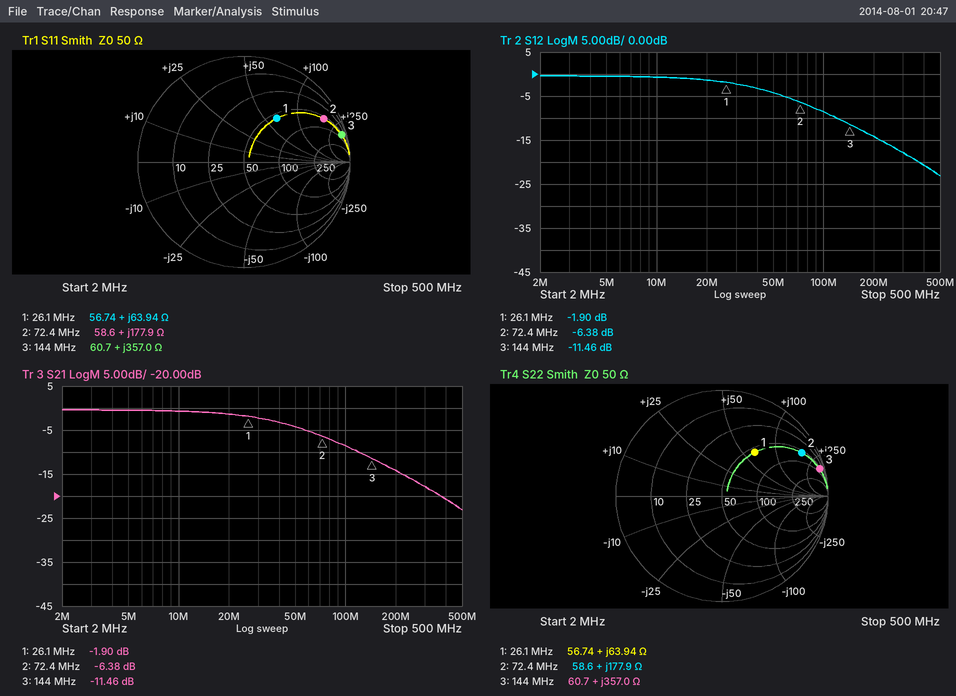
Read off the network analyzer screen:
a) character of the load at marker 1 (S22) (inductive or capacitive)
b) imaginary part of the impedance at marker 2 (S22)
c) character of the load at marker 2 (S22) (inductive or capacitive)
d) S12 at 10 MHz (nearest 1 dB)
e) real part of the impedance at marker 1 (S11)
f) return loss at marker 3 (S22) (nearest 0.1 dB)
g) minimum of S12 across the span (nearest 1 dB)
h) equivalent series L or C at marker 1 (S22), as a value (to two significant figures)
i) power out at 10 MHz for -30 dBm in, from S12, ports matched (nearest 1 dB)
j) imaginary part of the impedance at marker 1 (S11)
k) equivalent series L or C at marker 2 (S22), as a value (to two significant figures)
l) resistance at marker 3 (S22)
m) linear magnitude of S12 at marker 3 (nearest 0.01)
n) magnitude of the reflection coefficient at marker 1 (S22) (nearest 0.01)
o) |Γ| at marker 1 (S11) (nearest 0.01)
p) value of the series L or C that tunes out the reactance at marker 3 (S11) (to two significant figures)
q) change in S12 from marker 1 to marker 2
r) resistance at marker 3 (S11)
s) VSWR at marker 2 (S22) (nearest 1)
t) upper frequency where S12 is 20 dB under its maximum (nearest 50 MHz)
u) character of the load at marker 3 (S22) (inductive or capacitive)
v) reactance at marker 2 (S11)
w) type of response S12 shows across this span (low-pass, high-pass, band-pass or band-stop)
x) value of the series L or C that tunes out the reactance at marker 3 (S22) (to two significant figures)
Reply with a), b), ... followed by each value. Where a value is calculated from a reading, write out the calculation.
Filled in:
a) inductive
b) +177.9 Ω
c) inductive
d) -1 dB
e) 56.74 Ω
f) 0.4 dB
g) -23 dB
h) L = 63.94 Ω/(2π × 26.1 MHz) ≈ 390 nH
i) -30 dBm + (-1 dB) = -31 dBm
j) +63.94 Ω
k) L = 177.9 Ω/(2π × 72.4 MHz) ≈ 391 nH, so 390 nH to two significant figures
l) 60.7 Ω
m) 10^(-11.46/20) ≈ 0.27
n) 0.52
o) 0.52
p) C = 1/(2π × 144 MHz × 357 Ω) ≈ 3.1 pF
q) -6.38 − (-1.9) = -4.48 dB
r) 60.7 Ω
s) 13
t) 400 MHz
u) inductive
v) +177.9 Ω
w) low-pass
x) C = 1/(2π × 144 MHz × 357 Ω) ≈ 3.1 pF
